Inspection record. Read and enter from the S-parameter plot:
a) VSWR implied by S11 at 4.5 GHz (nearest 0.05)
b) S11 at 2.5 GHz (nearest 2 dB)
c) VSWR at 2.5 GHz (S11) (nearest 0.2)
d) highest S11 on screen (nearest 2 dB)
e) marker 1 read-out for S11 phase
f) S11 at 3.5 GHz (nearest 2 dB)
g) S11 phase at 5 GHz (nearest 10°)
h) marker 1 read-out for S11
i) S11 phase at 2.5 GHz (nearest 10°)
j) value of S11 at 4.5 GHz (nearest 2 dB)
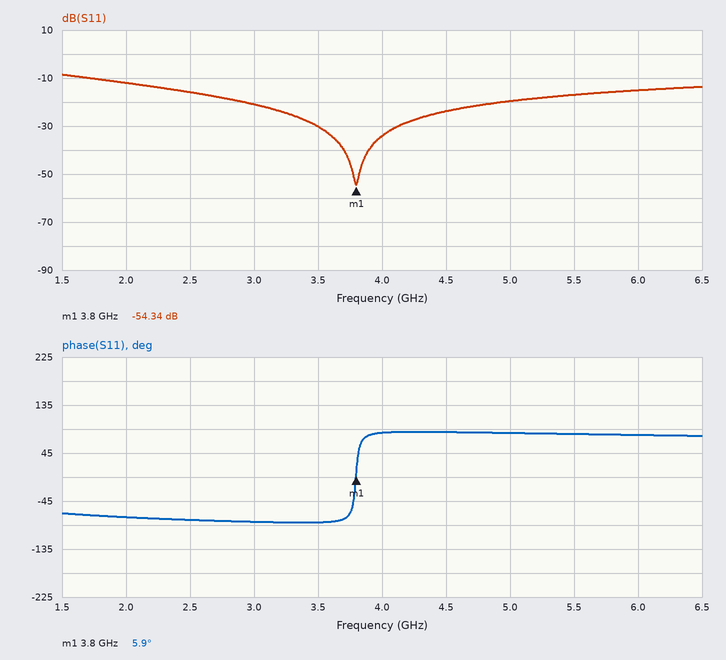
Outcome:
1.15
-16 dB
1.4
-8 dB
5.9°
-30 dB
80°
-54.34 dB
-80°
-24 dB
